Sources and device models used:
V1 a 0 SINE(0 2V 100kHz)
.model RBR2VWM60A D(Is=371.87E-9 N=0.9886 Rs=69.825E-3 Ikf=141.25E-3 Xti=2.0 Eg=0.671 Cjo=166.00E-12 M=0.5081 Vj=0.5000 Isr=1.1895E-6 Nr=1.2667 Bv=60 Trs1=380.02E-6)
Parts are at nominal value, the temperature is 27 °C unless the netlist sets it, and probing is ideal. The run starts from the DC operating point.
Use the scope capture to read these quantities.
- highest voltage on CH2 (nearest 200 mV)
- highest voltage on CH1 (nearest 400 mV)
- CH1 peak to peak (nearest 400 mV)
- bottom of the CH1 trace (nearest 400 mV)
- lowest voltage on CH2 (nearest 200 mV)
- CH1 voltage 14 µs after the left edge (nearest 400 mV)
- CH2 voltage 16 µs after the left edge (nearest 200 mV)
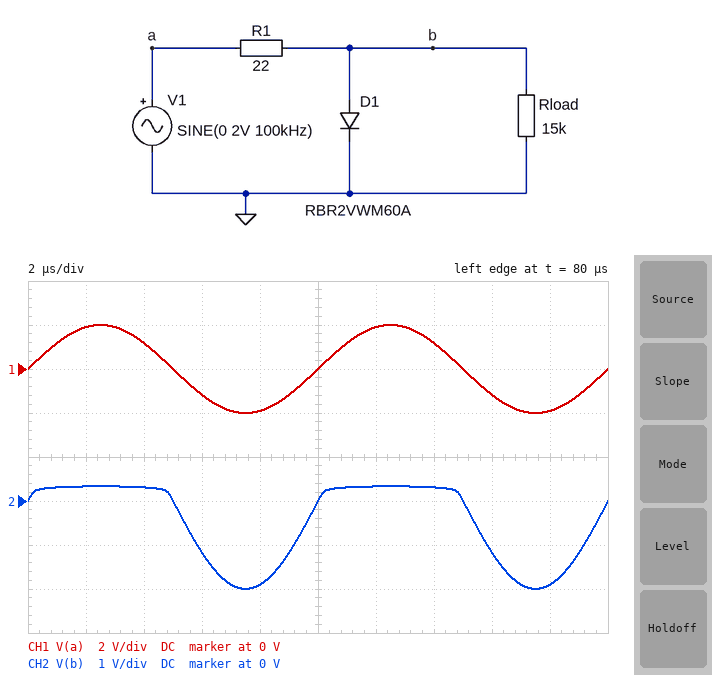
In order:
400 mV
2.0 V
4.0 V
-2.0 V
-2.0 V
1.2 V
-1.2 V
